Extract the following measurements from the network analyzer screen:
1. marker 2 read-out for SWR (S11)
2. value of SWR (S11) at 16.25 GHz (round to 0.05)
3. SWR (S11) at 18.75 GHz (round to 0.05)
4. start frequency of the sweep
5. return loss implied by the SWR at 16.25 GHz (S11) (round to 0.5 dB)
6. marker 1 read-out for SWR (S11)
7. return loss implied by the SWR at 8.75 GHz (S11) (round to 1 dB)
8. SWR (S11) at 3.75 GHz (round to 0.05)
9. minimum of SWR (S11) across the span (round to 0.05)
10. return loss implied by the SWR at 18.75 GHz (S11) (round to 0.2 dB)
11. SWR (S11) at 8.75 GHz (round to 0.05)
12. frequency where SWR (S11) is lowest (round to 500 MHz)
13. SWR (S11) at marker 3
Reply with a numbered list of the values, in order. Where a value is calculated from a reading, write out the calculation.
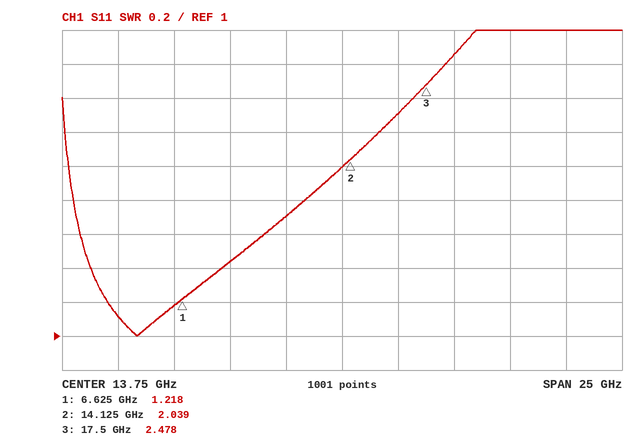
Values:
1. 2.039
2. 2.30
3. 2.65
4. 1.25 GHz
5. −20 log10((2.3 − 1)/(2.3 + 1)) ≈ 8.09 dB, so 8.0 dB to the nearest 0.5 dB
6. 1.218
7. −20 log10((1.45 − 1)/(1.45 + 1)) ≈ 15 dB
8. 1.10
9. 1.00
10. −20 log10((2.65 − 1)/(2.65 + 1)) ≈ 6.90 dB, so 6.8 dB to the nearest 0.2 dB
11. 1.45
12. 4.5 GHz
13. 2.478
